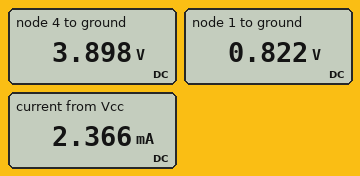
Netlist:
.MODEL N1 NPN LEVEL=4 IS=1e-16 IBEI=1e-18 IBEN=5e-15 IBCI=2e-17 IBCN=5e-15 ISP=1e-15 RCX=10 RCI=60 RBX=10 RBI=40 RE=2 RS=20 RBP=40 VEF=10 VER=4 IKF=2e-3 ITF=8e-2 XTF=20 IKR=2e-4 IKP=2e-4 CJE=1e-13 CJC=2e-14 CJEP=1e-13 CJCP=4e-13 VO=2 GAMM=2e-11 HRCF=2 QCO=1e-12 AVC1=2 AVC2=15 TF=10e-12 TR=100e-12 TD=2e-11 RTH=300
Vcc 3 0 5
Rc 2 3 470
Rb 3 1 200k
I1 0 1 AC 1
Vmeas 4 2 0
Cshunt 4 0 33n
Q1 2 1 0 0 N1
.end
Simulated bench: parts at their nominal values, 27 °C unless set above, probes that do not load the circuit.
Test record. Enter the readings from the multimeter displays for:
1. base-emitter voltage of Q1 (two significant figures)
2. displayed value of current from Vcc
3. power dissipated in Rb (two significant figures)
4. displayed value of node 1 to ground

820 mV
2.366 mA
87 µW
0.822 V
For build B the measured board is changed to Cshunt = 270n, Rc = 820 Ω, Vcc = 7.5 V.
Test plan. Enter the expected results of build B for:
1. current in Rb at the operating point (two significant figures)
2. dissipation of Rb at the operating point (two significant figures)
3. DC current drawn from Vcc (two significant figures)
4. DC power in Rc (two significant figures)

33 µA
220 µW
3.9 mA
12 mW
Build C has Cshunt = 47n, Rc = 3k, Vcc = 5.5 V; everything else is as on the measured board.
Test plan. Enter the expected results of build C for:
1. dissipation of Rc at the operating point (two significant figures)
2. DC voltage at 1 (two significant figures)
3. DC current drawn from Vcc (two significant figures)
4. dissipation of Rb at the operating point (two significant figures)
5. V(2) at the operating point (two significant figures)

4.8 mW
800 mV
1.3 mA
110 µW
1.7 V
